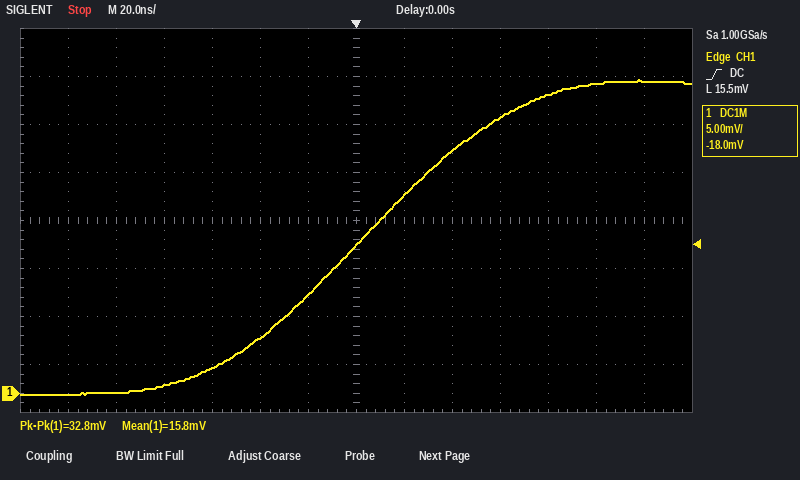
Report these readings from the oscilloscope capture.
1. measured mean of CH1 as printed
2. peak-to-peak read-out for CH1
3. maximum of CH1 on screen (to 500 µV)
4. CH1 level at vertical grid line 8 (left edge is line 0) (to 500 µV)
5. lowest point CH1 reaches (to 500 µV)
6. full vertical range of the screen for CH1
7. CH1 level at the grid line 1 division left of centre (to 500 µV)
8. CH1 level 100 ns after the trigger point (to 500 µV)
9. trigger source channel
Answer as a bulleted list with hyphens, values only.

- 15.8 mV
- 32.8 mV
- 32.5 mV
- 20.5 mV
- 0.0 mV
- 40 mV
- 10.5 mV
- 32.5 mV
- CH1
